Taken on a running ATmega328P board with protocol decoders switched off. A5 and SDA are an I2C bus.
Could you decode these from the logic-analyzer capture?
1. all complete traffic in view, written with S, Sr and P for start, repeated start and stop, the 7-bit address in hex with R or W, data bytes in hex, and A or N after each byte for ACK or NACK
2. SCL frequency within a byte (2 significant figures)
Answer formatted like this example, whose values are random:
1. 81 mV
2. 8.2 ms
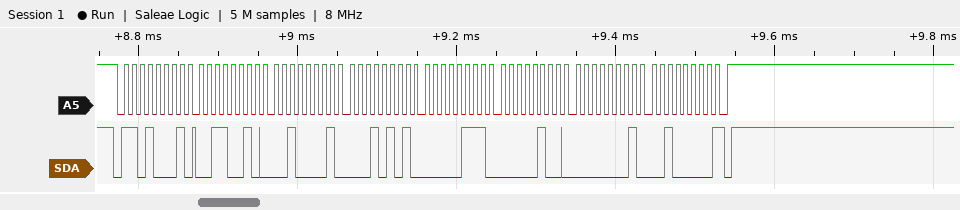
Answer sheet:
1. S 68R A 32 A 21 A 15 A 07 A 04 A 01 A 20 N P
2. 100 kHz
